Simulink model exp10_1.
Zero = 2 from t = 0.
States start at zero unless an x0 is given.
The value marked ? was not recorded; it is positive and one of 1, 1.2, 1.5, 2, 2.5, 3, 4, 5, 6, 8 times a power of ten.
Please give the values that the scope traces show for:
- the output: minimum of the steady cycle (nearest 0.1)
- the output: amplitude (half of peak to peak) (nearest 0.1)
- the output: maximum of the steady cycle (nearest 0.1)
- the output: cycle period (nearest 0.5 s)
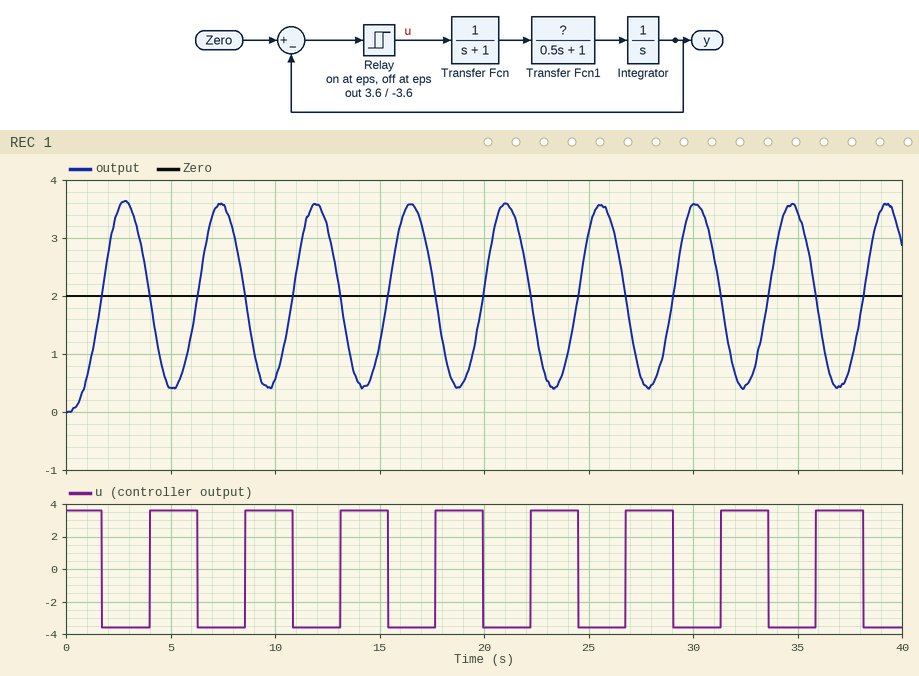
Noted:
0.4
1.6
3.6
4.5 s
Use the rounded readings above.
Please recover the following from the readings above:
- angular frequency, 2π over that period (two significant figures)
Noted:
1.4 rad/s
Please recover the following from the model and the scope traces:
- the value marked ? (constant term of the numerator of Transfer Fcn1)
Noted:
1
